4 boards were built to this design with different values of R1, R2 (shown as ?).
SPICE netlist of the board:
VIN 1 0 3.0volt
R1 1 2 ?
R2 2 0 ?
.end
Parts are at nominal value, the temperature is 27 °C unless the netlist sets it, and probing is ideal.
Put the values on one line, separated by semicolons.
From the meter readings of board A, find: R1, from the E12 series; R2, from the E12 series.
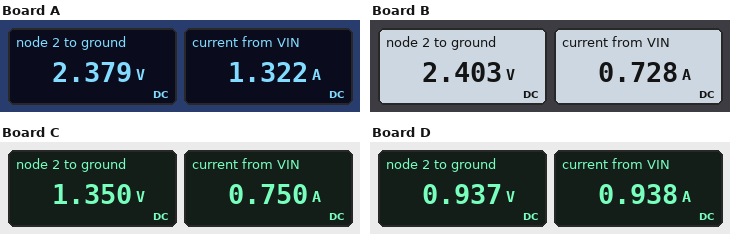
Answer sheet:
0.47 Ω; 1.8 Ω
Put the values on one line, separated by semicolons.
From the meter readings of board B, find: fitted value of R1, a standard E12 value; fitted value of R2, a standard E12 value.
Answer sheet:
0.82 Ω; 3.3 Ω
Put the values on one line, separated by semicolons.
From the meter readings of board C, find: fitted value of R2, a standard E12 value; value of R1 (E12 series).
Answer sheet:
1.8 Ω; 2.2 Ω
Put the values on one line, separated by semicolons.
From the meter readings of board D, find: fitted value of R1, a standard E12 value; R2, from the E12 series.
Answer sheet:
2.2 Ω; 1 Ω
